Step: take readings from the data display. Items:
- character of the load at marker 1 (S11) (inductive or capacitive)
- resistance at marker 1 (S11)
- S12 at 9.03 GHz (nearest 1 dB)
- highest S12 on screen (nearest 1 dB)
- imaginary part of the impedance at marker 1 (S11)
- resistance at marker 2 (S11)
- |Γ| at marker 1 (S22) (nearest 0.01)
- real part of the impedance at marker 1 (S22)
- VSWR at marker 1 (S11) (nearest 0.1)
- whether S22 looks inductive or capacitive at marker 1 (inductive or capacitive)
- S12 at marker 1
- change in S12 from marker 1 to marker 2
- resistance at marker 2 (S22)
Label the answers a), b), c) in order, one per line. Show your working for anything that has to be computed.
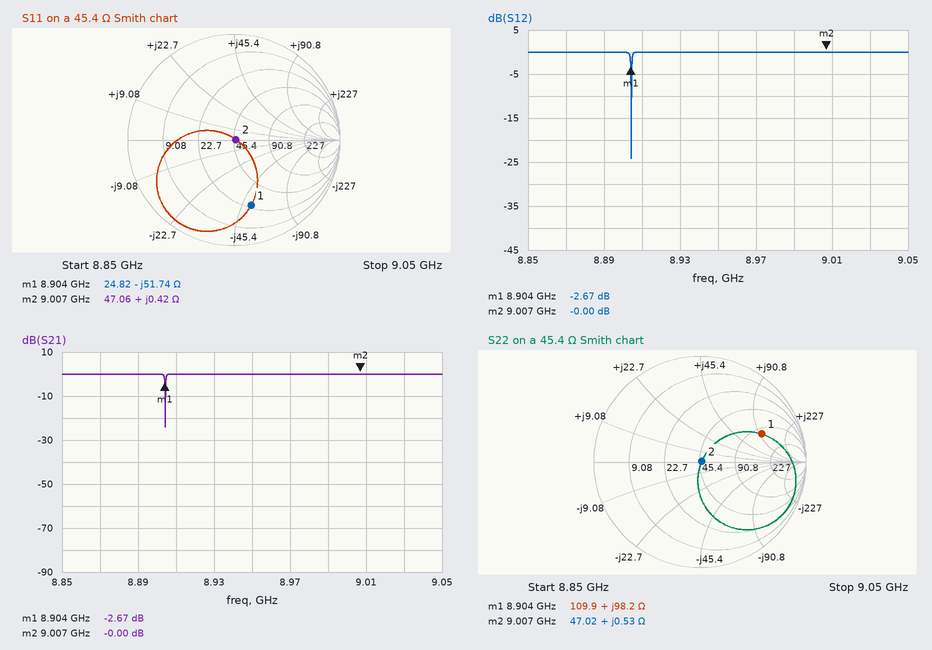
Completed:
a) capacitive
b) 24.82 Ω
c) 0 dB
d) 0 dB
e) -51.74 Ω
f) 47.06 Ω
g) 0.64
h) 109.9 Ω
i) 4.5
j) inductive
k) -2.67 dB
l) -0 − (-2.67) = 2.67 dB
m) 47.02 Ω
